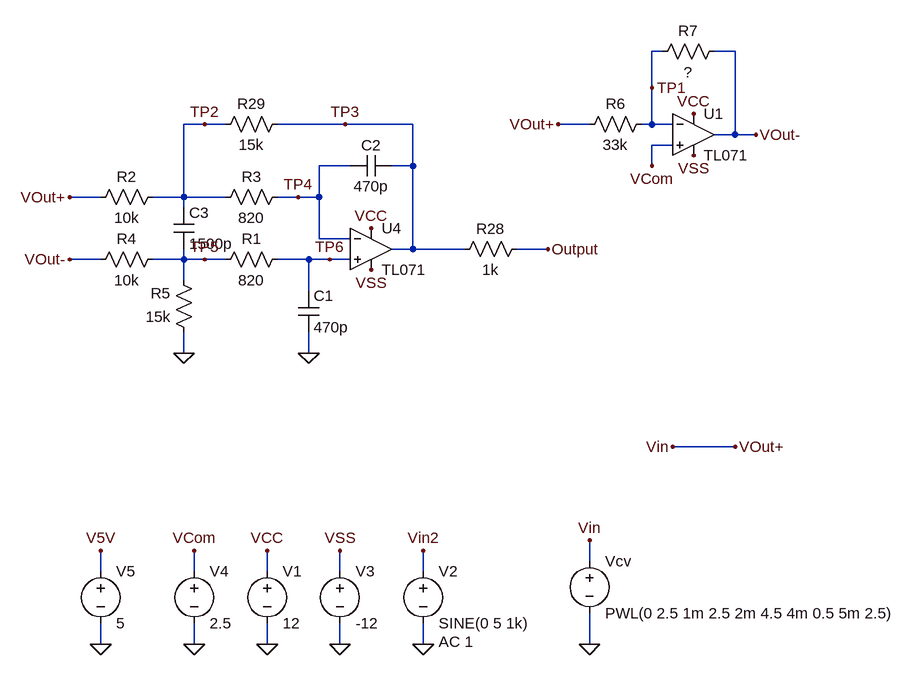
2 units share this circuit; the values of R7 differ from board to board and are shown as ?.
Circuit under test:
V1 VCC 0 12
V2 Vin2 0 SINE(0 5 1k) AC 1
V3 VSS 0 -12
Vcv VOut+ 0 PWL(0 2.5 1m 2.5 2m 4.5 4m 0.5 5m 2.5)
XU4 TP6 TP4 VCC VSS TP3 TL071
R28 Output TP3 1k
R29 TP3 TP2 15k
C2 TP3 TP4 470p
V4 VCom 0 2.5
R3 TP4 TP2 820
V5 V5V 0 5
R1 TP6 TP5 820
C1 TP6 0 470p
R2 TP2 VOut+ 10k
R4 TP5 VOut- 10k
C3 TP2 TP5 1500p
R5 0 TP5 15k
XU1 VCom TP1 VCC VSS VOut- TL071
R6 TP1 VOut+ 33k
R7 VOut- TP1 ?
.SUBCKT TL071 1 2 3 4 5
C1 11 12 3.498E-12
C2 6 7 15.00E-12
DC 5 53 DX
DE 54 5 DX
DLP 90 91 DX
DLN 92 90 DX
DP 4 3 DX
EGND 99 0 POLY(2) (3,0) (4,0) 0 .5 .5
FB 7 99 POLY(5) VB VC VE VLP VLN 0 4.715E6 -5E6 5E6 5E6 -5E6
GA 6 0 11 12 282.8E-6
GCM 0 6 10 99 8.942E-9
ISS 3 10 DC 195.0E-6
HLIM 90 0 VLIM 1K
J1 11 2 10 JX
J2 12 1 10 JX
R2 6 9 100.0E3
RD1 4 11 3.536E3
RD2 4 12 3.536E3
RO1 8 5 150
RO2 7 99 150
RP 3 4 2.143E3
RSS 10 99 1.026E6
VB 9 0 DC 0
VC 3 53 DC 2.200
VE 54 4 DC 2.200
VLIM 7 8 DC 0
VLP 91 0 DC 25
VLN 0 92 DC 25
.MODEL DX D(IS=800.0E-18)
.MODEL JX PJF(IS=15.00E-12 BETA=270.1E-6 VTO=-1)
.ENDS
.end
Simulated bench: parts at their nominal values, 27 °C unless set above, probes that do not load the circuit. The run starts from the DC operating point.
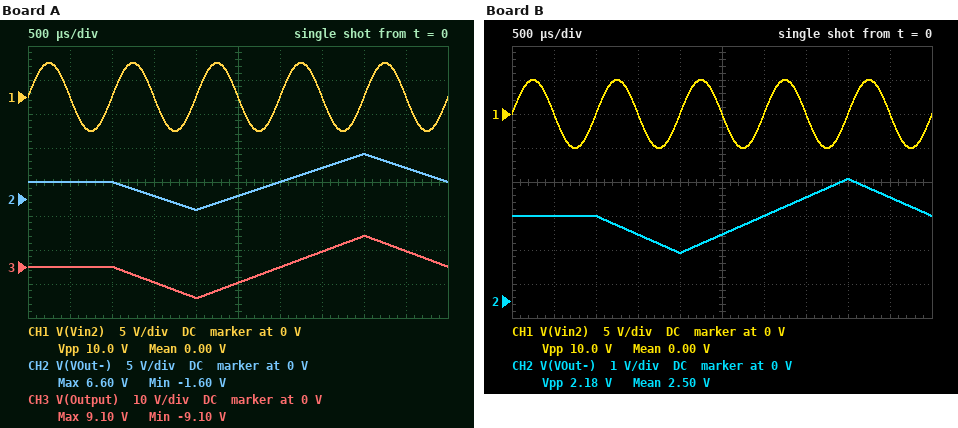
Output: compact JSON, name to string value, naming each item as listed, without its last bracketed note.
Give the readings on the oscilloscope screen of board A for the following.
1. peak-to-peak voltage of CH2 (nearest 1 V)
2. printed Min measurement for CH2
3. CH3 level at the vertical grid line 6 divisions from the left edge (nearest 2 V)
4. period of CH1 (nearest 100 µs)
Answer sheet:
{"peak-to-peak voltage of CH2": "8 V", "printed Min measurement for CH2": "-1.60 V", "CH3 level at the vertical grid line 6 divisions from the left edge": "0 V", "period of CH1": "1.0 ms"}
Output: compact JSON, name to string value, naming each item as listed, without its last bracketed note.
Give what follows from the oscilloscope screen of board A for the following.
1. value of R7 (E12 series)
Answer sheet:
{"value of R7": "68 kΩ"}
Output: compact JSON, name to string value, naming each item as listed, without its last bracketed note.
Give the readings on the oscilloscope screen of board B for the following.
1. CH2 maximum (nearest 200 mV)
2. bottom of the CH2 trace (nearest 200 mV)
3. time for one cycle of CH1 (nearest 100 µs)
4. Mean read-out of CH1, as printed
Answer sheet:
{"CH2 maximum": "3.6 V", "bottom of the CH2 trace": "1.4 V", "time for one cycle of CH1": "1.0 ms", "Mean read-out of CH1, as printed": "0.00 V"}
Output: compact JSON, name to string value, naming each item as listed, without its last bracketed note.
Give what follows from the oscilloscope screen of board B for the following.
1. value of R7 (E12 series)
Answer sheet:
{"value of R7": "18 kΩ"}
